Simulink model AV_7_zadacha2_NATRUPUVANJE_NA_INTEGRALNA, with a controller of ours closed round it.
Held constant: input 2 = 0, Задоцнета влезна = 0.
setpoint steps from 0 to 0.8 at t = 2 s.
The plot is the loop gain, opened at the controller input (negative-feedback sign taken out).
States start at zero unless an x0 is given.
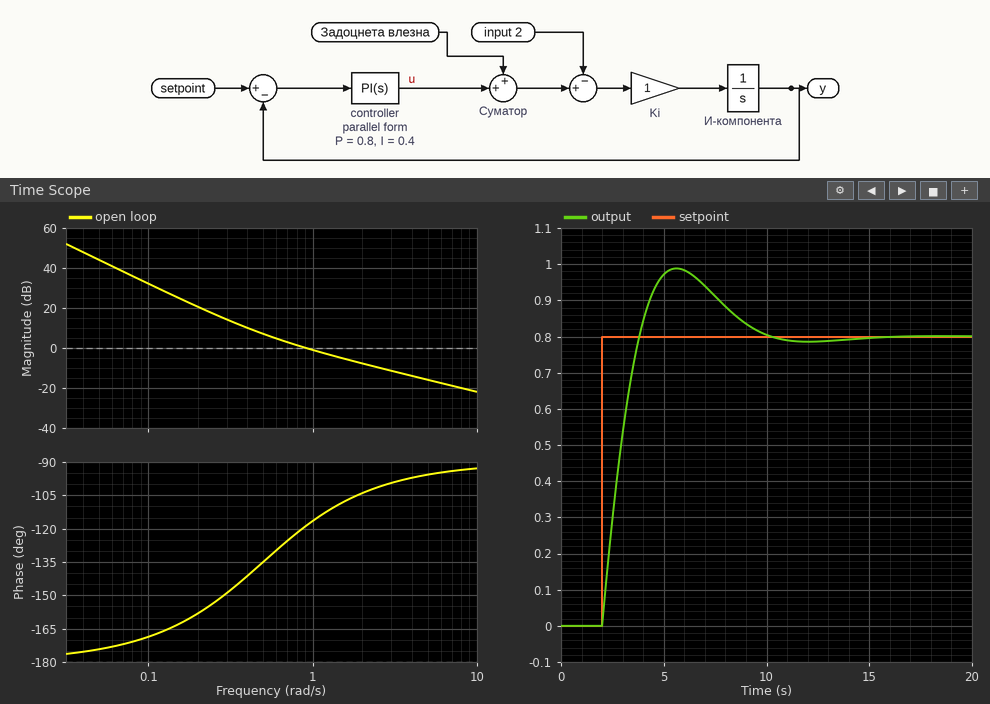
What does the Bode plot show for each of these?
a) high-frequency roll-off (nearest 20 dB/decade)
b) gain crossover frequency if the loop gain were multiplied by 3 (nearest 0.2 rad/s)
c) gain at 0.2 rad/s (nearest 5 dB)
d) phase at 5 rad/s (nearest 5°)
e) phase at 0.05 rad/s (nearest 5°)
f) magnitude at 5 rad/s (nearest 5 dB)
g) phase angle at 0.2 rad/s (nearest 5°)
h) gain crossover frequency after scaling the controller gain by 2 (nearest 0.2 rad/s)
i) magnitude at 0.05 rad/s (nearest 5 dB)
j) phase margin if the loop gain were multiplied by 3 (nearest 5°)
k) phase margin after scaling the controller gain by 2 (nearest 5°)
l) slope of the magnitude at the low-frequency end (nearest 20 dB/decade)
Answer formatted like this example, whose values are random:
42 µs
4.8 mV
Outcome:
-20 dB/decade
2.4 rad/s
20 dB
-95°
-175°
-15 dB
-160°
1.6 rad/s
45 dB
80°
75°
-40 dB/decade
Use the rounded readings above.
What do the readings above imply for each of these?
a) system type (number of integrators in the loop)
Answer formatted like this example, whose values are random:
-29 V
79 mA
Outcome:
2
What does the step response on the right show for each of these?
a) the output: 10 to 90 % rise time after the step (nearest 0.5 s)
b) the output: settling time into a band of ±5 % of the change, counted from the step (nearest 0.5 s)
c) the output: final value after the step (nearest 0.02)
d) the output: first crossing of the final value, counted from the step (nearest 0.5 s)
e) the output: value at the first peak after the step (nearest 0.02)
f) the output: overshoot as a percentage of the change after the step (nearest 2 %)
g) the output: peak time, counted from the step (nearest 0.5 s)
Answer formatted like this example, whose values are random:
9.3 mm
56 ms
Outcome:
1.5 s
7.0 s
0.80
2.0 s
0.98
24 %
3.5 s
